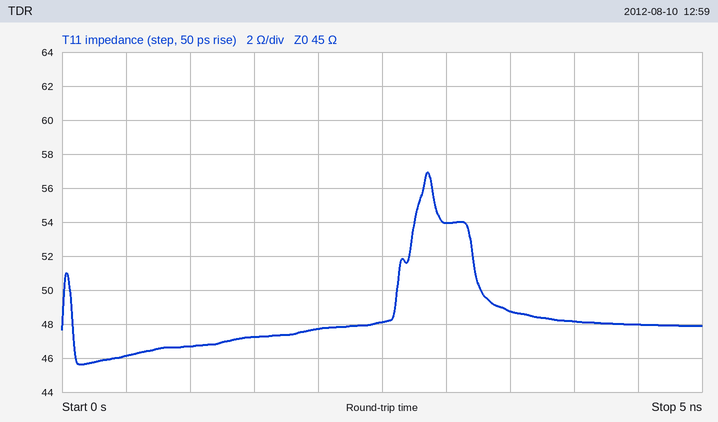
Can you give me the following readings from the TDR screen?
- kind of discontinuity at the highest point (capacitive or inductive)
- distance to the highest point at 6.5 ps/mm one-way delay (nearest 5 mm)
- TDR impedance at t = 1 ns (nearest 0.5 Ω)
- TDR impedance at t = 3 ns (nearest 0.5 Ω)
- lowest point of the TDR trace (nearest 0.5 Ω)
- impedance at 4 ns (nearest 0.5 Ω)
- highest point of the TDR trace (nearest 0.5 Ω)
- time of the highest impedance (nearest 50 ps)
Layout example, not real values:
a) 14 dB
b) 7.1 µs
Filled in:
a) inductive
b) 220 mm
c) 46.5 Ω
d) 54.0 Ω
e) 45.5 Ω
f) 48.0 Ω
g) 57.0 Ω
h) 2.85 ns
